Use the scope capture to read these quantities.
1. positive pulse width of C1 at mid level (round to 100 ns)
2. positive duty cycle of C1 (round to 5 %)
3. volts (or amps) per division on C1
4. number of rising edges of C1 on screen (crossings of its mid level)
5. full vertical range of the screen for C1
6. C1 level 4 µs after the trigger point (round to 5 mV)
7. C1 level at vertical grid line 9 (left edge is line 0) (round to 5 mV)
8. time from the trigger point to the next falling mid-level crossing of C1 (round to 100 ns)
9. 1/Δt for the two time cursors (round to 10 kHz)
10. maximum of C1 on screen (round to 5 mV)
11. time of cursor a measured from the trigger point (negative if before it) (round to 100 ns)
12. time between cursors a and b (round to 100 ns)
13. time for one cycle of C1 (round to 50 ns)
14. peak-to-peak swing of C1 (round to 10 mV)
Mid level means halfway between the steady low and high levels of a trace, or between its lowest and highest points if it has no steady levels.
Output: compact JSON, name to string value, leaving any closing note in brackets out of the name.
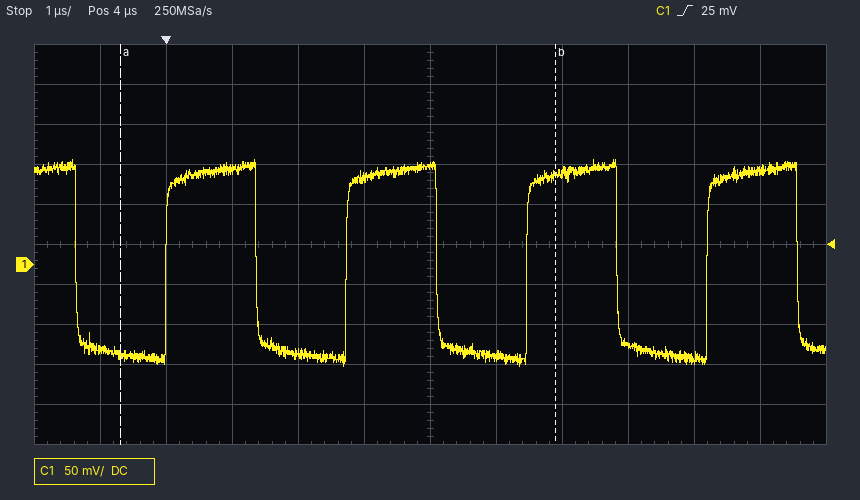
{"positive pulse width of C1 at mid level": "1.4 µs", "positive duty cycle of C1": "50 %", "volts (or amps) per division on C1": "50 mV", "number of rising edges of C1 on screen": "4", "full vertical range of the screen for C1": "500 mV", "C1 level 4 µs after the trigger point": "125 mV", "C1 level at vertical grid line 9 (left edge is line 0)": "-100 mV", "time from the trigger point to the next falling mid-level crossing of C1": "1.4 µs", "1/Δt for the two time cursors": "150 kHz", "maximum of C1 on screen": "130 mV", "time of cursor a measured from the trigger point (negative if before it)": "-700 ns", "time between cursors a and b": "6.6 µs", "time for one cycle of C1": "2.75 µs", "peak-to-peak swing of C1": "260 mV"}
